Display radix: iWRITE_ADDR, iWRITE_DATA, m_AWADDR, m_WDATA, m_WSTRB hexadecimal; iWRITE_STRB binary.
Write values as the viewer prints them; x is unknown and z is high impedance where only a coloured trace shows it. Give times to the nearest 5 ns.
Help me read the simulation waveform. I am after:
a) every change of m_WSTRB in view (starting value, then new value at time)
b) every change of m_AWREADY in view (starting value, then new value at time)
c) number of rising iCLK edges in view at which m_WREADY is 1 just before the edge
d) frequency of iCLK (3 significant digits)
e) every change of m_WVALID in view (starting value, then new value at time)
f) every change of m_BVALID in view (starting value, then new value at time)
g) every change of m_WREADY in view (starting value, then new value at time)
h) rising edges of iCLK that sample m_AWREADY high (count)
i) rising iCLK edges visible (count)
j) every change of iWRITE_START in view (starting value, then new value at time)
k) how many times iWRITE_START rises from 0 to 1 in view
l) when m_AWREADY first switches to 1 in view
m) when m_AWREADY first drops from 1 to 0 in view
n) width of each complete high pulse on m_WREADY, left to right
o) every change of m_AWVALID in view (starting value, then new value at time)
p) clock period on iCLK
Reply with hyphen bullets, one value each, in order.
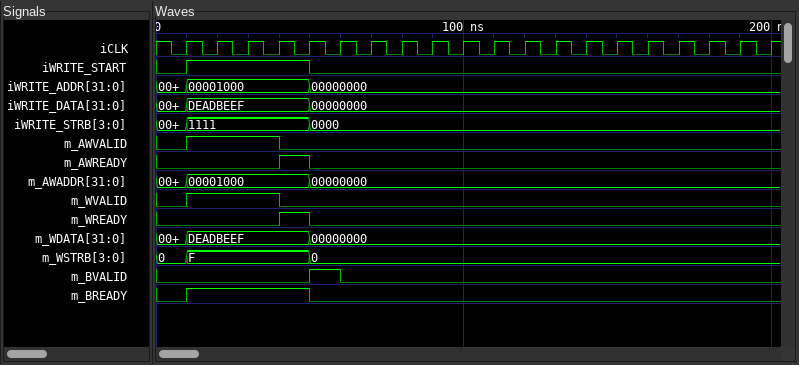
- 0, F at 10 ns, 0 at 50 ns
- 0, 1 at 40 ns, 0 at 50 ns
- 1
- 100 MHz
- 0, 1 at 10 ns, 0 at 40 ns
- 0, 1 at 50 ns, 0 at 60 ns
- 0, 1 at 40 ns, 0 at 50 ns
- 1
- 20
- 0, 1 at 10 ns, 0 at 50 ns
- 1
- 40 ns
- 50 ns
- 10 ns
- 0, 1 at 10 ns, 0 at 40 ns
- 10 ns
